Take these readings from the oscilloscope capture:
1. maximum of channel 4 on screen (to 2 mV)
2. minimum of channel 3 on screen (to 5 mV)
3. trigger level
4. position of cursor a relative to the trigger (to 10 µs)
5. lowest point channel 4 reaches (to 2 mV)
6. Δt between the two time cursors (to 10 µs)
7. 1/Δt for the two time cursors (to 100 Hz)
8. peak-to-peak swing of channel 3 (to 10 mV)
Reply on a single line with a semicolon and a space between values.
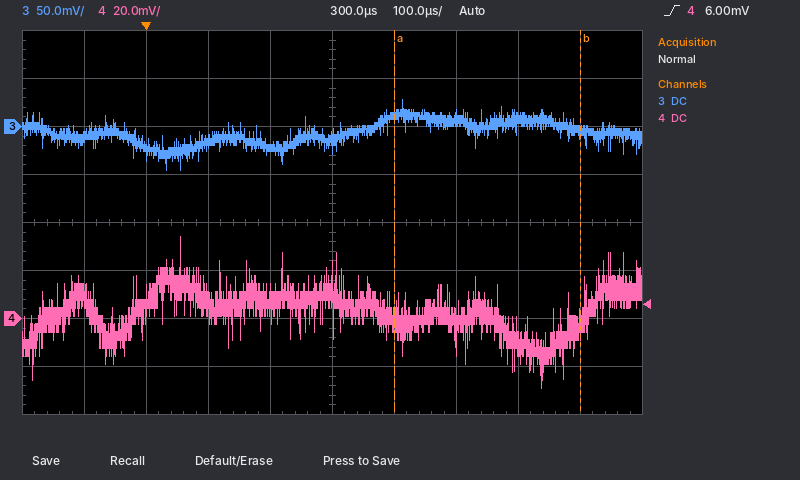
34 mV; -45 mV; 6.00 mV; +400 µs; -28 mV; 300 µs; 3.3 kHz; 70 mV
